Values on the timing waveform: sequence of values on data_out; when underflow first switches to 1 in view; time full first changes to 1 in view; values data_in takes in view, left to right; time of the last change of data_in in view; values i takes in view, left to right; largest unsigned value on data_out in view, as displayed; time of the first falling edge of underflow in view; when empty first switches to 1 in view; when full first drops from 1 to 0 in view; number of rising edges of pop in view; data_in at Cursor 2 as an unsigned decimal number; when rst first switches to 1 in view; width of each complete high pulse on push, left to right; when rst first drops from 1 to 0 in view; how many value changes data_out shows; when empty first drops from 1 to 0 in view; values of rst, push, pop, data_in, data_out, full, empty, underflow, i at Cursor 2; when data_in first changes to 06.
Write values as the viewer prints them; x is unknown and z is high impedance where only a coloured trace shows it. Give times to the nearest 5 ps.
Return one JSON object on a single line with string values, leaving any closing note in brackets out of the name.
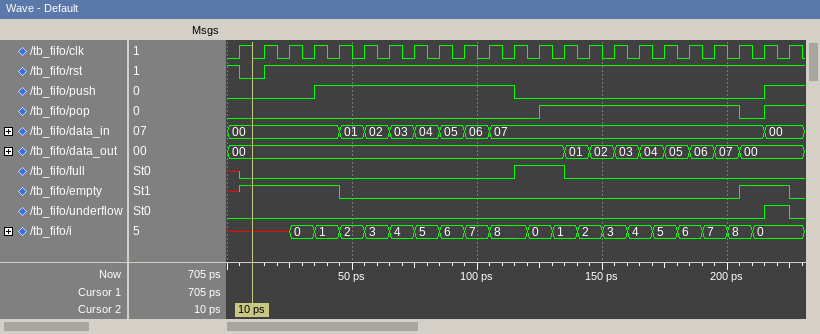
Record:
{"sequence of values on data_out": "00, 01, 02, 03, 04, 05, 06, 07, 00", "when underflow first switches to 1 in view": "215 ps", "time full first changes to 1 in view": "115 ps", "values data_in takes in view, left to right": "00, 01, 02, 03, 04, 05, 06, 07, 00", "time of the last change of data_in in view": "215 ps", "values i takes in view, left to right": "x, 0, 1, 2, 3, 4, 5, 6, 7, 8, 0, 1, 2, 3, 4, 5, 6, 7, 8, 0", "largest unsigned value on data_out in view, as displayed": "07", "time of the first falling edge of underflow in view": "225 ps", "when empty first switches to 1 in view": "5 ps", "when full first drops from 1 to 0 in view": "135 ps", "number of rising edges of pop in view": "2", "data_in at Cursor 2 as an unsigned decimal number": "0", "when rst first switches to 1 in view": "15 ps", "width of each complete high pulse on push, left to right": "80 ps", "when rst first drops from 1 to 0 in view": "5 ps", "how many value changes data_out shows": "8", "when empty first drops from 1 to 0 in view": "45 ps", "values of rst, push, pop, data_in, data_out, full, empty, underflow, i at Cursor 2": "rst=0, push=0, pop=0, data_in=00, data_out=00, full=0, empty=1, underflow=0, i=x", "when data_in first changes to 06": "95 ps"}
